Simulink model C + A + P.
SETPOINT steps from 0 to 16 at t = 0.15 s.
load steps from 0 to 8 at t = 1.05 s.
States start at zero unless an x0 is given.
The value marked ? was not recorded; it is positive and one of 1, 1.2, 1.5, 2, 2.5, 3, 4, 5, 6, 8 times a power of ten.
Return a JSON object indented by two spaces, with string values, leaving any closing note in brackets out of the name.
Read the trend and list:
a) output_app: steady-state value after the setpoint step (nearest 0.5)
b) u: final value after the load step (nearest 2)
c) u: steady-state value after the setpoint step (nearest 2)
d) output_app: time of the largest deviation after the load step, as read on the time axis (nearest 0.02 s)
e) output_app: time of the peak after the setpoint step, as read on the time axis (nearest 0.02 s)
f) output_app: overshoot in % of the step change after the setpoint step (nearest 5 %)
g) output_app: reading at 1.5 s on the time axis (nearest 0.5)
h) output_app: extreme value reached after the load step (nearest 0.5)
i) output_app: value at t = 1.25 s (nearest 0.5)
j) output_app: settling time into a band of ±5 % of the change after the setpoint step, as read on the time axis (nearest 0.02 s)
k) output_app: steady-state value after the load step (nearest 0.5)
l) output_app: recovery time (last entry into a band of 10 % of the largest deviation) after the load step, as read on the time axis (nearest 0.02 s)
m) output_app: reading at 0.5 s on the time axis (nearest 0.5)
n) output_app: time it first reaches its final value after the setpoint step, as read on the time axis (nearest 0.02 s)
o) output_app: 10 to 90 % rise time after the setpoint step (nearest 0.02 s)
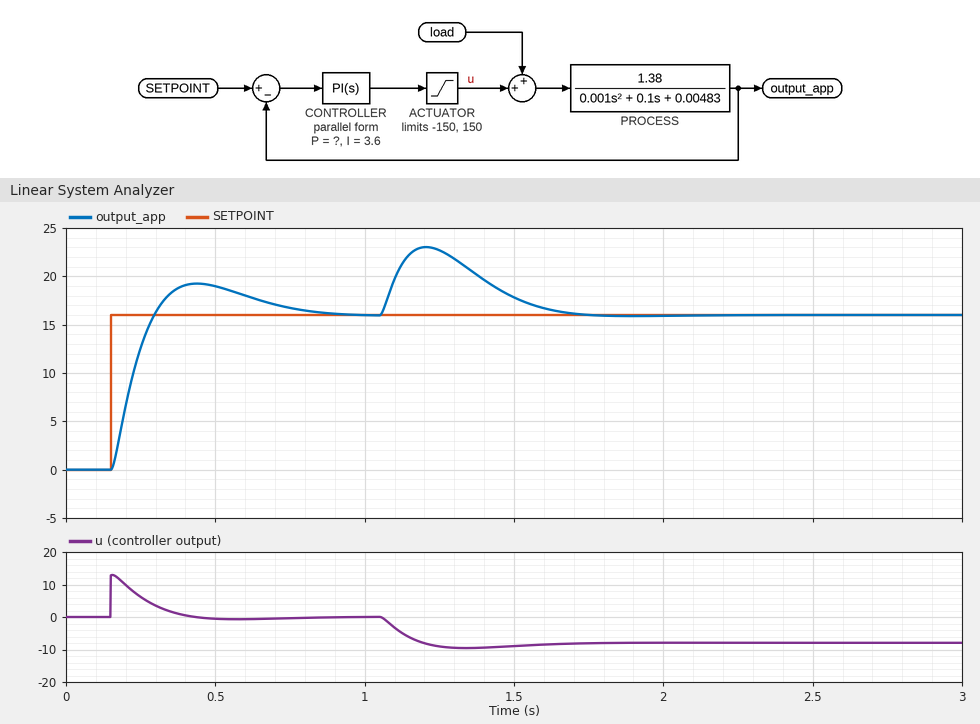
{
  "output_app: steady-state value after the setpoint step": "16.0",
  "u: final value after the load step": "-8",
  "u: steady-state value after the setpoint step": "0",
  "output_app: time of the largest deviation after the load step, as read on the time axis": "1.20 s",
  "output_app: time of the peak after the setpoint step, as read on the time axis": "0.44 s",
  "output_app: overshoot in % of the step change after the setpoint step": "20 %",
  "output_app: reading at 1.5 s on the time axis": "18.0",
  "output_app: extreme value reached after the load step": "23.0",
  "output_app: value at t = 1.25 s": "22.5",
  "output_app: settling time into a band of ±5 % of the change after the setpoint step, as read on the time axis": "0.74 s",
  "output_app: steady-state value after the load step": "16.0",
  "output_app: recovery time (last entry into a band of 10 % of the largest deviation) after the load step, as read on the time axis": "1.60 s",
  "output_app: reading at 0.5 s on the time axis": "19.0",
  "output_app: time it first reaches its final value after the setpoint step, as read on the time axis": "0.30 s",
  "output_app: 10 to 90 % rise time after the setpoint step": "0.10 s"
}
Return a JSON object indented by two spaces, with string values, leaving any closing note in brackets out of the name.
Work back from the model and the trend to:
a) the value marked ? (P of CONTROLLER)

{
  "the value marked ?": "0.8"
}
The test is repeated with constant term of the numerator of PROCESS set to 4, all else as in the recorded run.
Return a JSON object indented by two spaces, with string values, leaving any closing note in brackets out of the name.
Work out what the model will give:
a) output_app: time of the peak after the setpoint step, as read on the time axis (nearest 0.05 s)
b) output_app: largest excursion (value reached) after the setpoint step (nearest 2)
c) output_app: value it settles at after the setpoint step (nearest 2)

{
  "output_app: time of the peak after the setpoint step, as read on the time axis": "0.25 s",
  "output_app: largest excursion (value reached) after the setpoint step": "18",
  "output_app: value it settles at after the setpoint step": "16"
}
